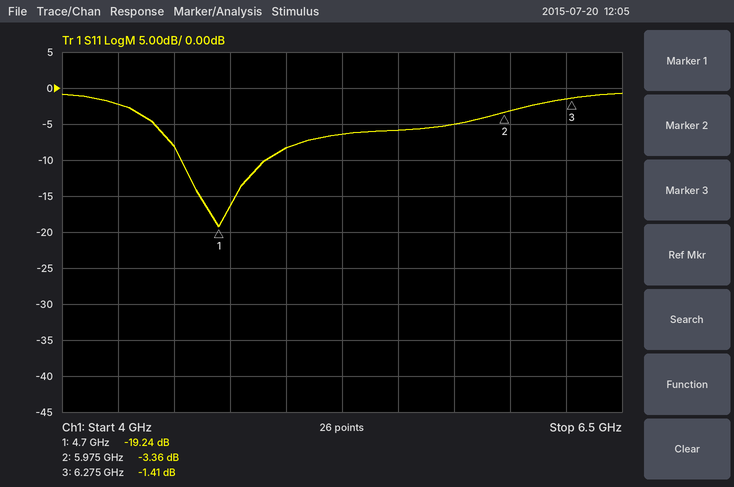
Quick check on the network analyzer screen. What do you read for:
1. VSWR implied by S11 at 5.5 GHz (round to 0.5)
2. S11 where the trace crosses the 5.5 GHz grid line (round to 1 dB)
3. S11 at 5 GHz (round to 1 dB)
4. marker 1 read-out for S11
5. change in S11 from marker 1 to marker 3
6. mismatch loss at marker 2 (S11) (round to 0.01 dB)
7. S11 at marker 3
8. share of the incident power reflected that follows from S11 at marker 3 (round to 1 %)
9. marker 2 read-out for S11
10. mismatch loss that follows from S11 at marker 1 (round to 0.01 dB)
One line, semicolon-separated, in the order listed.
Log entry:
3.0; -6 dB; -8 dB; -19.24 dB; 17.83 dB; 2.69 dB; -1.41 dB; 72 %; -3.36 dB; 0.05 dB
